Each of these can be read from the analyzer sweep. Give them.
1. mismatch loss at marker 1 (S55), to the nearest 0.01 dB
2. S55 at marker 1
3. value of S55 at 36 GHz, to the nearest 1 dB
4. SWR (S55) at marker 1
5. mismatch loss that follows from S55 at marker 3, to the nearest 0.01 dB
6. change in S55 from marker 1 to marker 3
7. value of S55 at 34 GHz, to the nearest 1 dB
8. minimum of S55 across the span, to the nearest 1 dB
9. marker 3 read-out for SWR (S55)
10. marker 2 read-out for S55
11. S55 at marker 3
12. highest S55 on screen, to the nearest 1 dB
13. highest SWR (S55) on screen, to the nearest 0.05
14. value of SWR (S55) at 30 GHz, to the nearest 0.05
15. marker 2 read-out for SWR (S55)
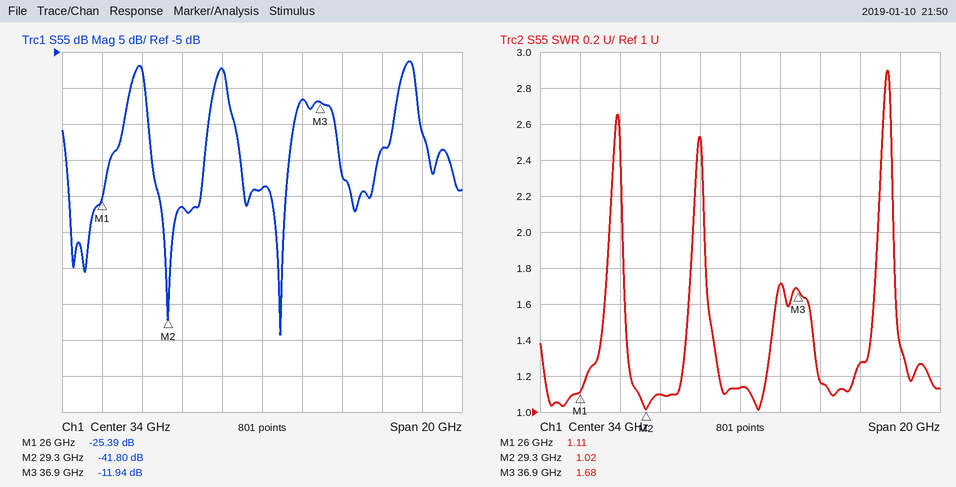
0.01 dB
-25.39 dB
-12 dB
1.11
0.29 dB
13.45 dB
-24 dB
-44 dB
1.68
-41.80 dB
-11.94 dB
-6 dB
2.90
1.10
1.02
